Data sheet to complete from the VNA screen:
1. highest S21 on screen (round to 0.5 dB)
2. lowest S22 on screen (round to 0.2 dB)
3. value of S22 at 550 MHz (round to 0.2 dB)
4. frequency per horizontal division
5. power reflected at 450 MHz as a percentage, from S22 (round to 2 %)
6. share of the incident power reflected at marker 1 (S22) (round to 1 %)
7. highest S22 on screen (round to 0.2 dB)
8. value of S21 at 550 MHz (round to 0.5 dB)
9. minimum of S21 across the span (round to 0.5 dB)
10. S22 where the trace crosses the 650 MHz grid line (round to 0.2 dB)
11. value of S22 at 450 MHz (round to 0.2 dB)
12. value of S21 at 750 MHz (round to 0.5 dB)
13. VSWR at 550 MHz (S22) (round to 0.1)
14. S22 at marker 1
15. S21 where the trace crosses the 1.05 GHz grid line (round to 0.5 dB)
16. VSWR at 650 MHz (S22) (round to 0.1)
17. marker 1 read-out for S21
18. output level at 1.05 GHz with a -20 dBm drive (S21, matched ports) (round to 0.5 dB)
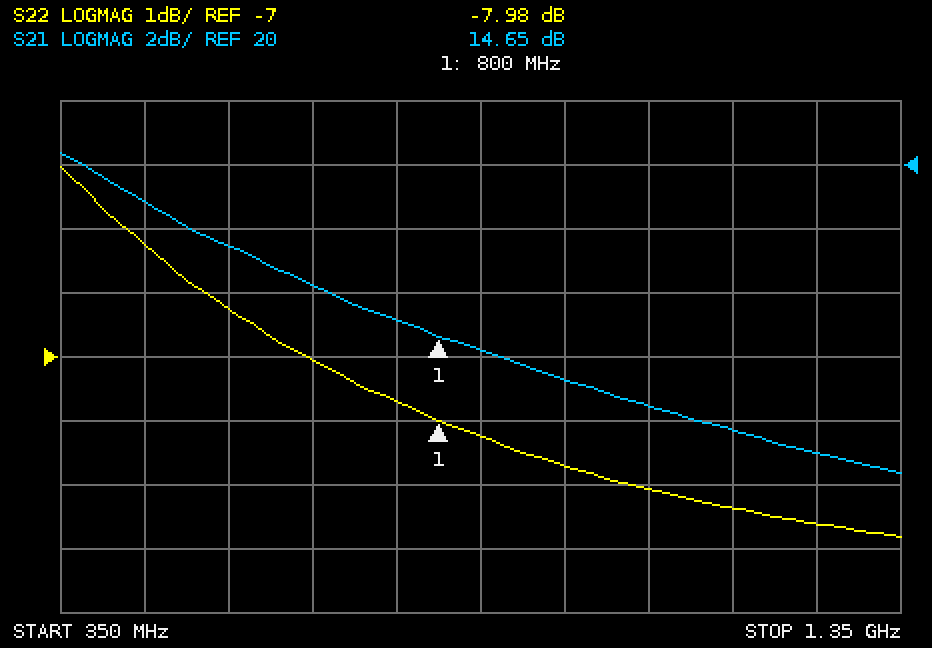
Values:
20.5 dB
-9.8 dB
-6.2 dB
100 MHz
30 %
16 %
-4.0 dB
17.5 dB
10.5 dB
-7.0 dB
-5.2 dB
15.0 dB
2.9
-7.98 dB
12.5 dB
2.6
14.65 dB
-7.5 dBm
